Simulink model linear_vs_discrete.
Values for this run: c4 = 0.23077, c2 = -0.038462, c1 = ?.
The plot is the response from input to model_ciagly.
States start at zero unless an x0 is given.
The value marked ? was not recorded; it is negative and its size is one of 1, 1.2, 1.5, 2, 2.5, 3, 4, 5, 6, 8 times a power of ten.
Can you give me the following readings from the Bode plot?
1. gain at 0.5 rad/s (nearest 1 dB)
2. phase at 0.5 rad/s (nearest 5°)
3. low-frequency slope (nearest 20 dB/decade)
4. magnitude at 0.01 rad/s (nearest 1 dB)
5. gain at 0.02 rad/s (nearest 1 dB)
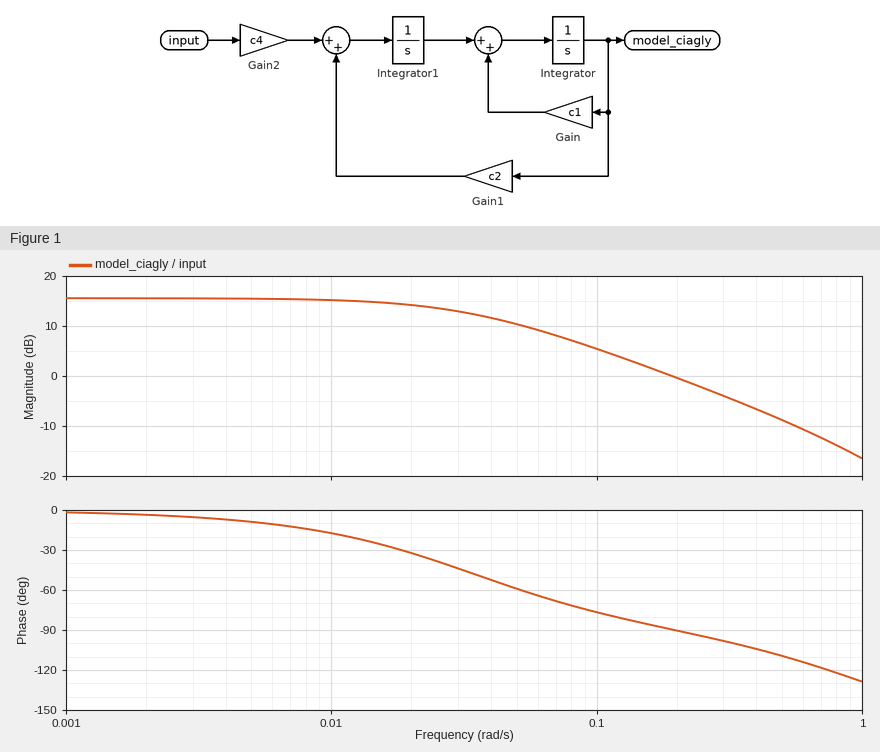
-9 dB
-110°
0 dB/decade
15 dB
14 dB
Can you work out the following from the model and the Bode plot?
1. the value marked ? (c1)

-1.2
